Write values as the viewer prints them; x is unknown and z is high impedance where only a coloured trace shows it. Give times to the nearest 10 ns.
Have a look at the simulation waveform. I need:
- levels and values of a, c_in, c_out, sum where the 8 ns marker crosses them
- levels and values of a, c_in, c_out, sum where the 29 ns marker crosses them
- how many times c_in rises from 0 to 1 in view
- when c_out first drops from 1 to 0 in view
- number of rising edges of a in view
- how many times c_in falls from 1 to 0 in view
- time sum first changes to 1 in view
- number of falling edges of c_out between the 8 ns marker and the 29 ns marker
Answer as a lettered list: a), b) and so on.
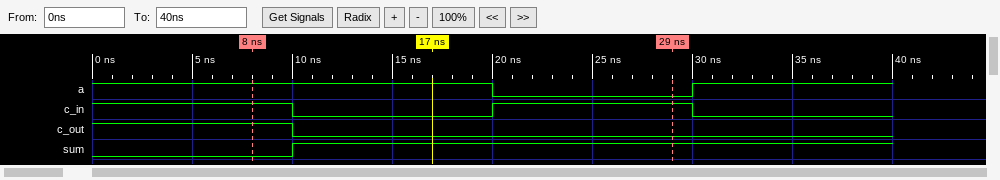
a) a=1, c_in=1, c_out=1, sum=0
b) a=0, c_in=1, c_out=0, sum=1
c) 1
d) 10 ns
e) 1
f) 2
g) 10 ns
h) 1
